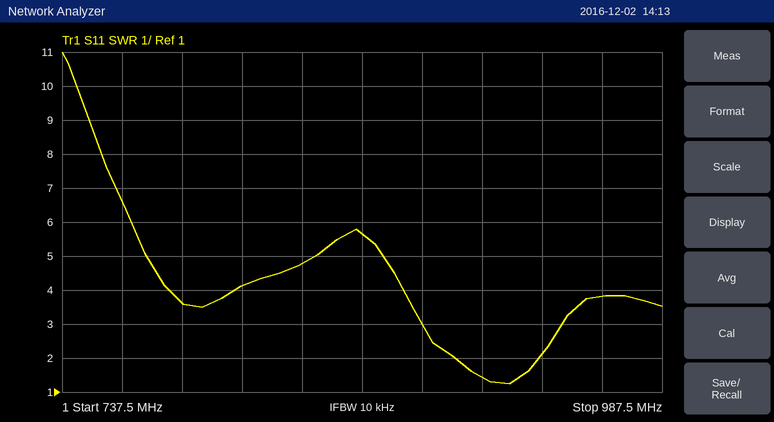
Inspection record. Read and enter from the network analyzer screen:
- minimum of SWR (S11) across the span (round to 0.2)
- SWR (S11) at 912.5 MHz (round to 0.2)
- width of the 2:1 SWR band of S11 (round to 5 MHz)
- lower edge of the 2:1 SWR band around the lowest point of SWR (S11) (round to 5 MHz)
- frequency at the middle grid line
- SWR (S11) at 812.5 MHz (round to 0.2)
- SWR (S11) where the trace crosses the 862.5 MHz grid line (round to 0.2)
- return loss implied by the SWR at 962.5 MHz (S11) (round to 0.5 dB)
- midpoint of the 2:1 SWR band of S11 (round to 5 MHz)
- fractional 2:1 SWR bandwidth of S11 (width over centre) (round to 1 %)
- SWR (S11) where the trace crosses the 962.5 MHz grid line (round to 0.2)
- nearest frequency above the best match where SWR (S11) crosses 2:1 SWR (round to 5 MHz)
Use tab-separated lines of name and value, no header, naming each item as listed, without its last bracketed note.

minimum of SWR (S11) across the span	1.2
SWR (S11) at 912.5 MHz	1.4
width of the 2:1 SWR band of S11	35 MHz
lower edge of the 2:1 SWR band around the lowest point of SWR (S11)	900 MHz
frequency at the middle grid line	862.5 MHz
SWR (S11) at 812.5 MHz	4.2
SWR (S11) where the trace crosses the 862.5 MHz grid line	5.6
return loss implied by the SWR at 962.5 MHz (S11)	4.5 dB
midpoint of the 2:1 SWR band of S11	920 MHz
fractional 2:1 SWR bandwidth of S11 (width over centre)	4 %
SWR (S11) where the trace crosses the 962.5 MHz grid line	3.8
nearest frequency above the best match where SWR (S11) crosses 2:1 SWR	935 MHz
